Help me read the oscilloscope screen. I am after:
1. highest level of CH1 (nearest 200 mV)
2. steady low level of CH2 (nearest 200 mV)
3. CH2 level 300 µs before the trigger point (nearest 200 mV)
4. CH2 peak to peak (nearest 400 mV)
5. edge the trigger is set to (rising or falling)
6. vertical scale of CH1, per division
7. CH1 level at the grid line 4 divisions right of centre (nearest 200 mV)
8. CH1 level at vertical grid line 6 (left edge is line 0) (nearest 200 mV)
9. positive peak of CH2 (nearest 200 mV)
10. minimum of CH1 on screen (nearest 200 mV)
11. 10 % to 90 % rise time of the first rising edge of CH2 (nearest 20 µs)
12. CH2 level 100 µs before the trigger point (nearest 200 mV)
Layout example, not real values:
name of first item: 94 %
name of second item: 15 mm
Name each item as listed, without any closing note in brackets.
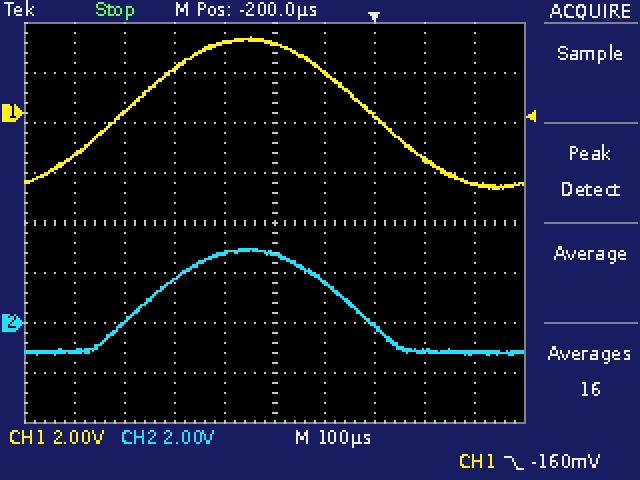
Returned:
highest level of CH1: 3.0 V
steady low level of CH2: -1.2 V
CH2 level 300 µs before the trigger point: 2.8 V
CH2 peak to peak: 4.4 V
edge the trigger is set to: falling
vertical scale of CH1, per division: 2 V
CH1 level at the grid line 4 divisions right of centre: -2.8 V
CH1 level at vertical grid line 6 (left edge is line 0): 1.6 V
positive peak of CH2: 3.0 V
minimum of CH1 on screen: -3.0 V
10 % to 90 % rise time of the first rising edge of CH2: 200 µs
CH2 level 100 µs before the trigger point: 1.6 V
